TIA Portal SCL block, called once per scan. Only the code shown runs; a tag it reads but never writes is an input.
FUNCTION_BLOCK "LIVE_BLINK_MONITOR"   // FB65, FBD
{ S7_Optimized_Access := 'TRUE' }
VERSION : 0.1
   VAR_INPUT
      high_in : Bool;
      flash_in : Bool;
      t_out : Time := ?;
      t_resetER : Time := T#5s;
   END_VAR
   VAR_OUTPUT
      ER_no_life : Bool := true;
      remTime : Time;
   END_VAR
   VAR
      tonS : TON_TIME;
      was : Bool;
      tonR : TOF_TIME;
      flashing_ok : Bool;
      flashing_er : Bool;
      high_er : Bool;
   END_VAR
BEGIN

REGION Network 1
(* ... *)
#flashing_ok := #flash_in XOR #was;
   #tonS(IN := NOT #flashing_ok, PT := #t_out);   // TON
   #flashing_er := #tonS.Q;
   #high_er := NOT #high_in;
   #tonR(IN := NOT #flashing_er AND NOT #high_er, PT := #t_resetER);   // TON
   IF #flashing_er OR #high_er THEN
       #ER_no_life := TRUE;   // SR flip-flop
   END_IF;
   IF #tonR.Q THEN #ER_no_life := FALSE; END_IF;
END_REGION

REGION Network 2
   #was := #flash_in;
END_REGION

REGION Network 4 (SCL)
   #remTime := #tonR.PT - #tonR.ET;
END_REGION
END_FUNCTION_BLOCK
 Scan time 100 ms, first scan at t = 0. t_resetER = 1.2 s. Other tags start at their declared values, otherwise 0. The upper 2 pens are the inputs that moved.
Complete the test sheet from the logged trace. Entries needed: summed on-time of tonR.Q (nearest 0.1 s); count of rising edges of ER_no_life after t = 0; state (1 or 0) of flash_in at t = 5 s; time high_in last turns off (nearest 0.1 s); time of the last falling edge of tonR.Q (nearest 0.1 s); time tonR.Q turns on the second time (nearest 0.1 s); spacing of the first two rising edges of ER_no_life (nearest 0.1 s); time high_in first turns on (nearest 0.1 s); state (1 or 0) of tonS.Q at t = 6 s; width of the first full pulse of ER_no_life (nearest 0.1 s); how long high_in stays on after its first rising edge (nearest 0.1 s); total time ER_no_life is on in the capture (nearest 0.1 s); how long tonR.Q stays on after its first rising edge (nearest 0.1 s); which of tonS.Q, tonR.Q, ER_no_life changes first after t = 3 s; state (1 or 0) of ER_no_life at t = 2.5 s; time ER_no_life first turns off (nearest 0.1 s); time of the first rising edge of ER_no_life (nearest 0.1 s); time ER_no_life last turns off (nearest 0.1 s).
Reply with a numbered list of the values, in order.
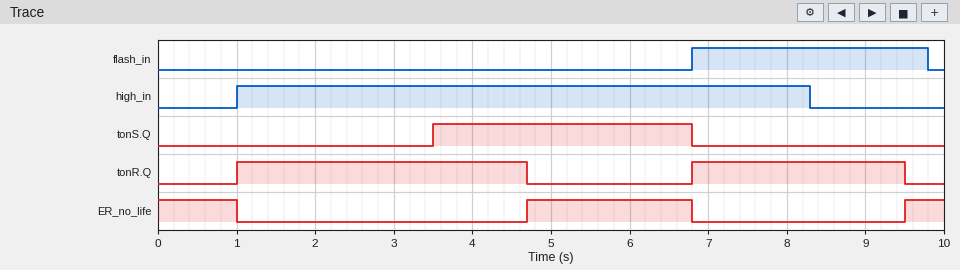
1. 6.4 s
2. 2
3. 0
4. 8.3 s
5. 9.5 s
6. 6.8 s
7. 4.8 s
8. 1.0 s
9. 1
10. 2.1 s
11. 7.3 s
12. 3.6 s
13. 3.7 s
14. tonS.Q
15. 0
16. 1.0 s
17. 4.7 s
18. 6.8 s
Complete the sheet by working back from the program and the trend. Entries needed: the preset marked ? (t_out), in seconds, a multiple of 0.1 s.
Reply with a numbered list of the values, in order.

1. 3.5 s
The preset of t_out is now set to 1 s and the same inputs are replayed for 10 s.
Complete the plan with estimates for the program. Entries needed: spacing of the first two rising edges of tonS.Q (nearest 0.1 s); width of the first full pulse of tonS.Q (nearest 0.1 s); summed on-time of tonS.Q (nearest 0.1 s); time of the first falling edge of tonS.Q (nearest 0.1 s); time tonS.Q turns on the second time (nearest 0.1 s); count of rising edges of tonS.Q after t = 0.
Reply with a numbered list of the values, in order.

1. 6.9 s
2. 5.8 s
3. 7.7 s
4. 6.8 s
5. 7.9 s
6. 2
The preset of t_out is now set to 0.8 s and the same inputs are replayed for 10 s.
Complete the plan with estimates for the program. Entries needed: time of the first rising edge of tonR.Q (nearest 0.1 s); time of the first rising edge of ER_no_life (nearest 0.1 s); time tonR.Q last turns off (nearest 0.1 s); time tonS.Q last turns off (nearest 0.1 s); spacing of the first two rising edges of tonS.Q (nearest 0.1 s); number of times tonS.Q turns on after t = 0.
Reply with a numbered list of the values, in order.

1. 6.8 s
2. 8.9 s
3. 8.9 s
4. 9.8 s
5. 6.9 s
6. 2
